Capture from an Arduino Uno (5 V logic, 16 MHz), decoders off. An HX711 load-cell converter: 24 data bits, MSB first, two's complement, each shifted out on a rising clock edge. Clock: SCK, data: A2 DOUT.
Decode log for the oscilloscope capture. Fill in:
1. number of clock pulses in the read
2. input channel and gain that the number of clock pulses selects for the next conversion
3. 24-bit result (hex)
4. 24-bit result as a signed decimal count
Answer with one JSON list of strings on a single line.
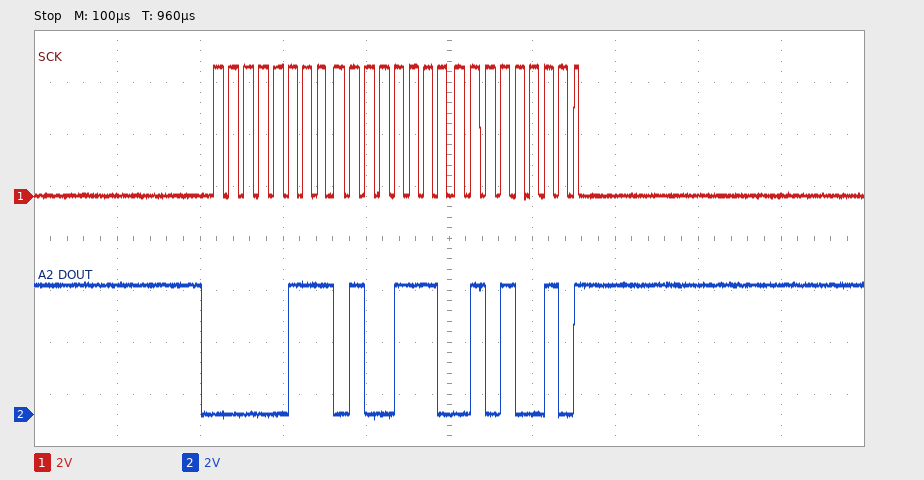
["25", "channel A, gain 128", "0x074E52", "478802"]
